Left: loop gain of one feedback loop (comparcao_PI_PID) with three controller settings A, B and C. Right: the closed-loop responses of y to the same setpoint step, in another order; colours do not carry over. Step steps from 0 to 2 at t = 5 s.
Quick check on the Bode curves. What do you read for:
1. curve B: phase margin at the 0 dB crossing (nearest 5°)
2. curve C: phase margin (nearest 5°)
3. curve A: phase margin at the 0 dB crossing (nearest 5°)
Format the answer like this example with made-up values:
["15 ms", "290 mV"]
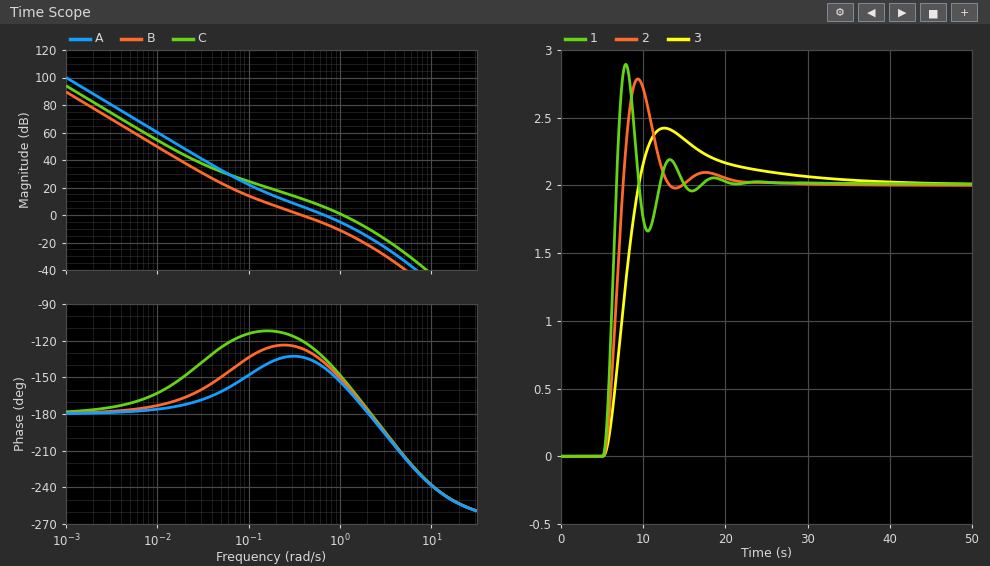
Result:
["55°", "30°", "40°"]
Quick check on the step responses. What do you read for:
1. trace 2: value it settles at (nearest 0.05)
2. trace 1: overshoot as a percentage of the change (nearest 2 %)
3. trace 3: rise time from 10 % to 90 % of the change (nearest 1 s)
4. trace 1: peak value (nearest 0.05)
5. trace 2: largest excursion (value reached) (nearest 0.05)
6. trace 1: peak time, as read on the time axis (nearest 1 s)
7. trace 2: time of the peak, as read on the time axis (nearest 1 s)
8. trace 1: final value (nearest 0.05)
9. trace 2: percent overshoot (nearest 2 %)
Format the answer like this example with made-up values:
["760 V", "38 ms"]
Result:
["2.00", "44 %", "3 s", "2.90", "2.80", "8 s", "9 s", "2.00", "40 %"]
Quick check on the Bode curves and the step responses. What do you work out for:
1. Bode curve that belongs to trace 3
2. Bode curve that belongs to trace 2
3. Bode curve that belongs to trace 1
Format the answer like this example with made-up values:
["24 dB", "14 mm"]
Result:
["B", "A", "C"]
